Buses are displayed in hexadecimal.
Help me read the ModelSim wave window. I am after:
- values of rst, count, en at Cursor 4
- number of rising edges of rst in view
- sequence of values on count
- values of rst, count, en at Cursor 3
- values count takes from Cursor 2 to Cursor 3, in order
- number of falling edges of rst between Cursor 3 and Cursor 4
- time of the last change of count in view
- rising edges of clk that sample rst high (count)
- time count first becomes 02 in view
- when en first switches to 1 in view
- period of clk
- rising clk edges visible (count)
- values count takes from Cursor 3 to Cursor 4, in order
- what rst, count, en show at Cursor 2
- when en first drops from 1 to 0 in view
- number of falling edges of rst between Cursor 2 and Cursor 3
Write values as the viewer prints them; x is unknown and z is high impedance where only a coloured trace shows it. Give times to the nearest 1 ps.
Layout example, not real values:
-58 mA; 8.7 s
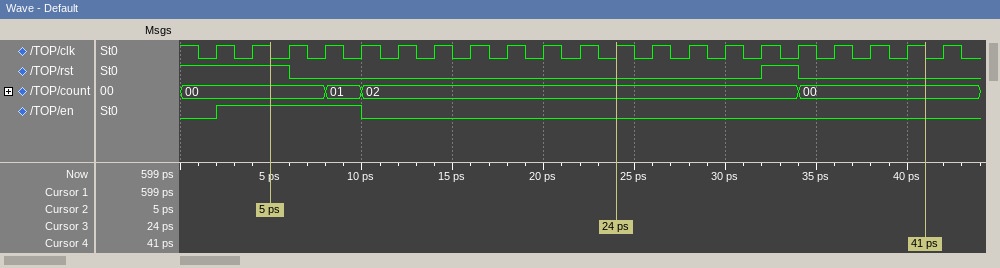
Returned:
rst=0, count=00, en=0; 1; 00, 01, 02, 00; rst=0, count=02, en=0; 00, 01, 02; 1; 34 ps; 4; 10 ps; 2 ps; 2 ps; 21; 02, 00; rst=1, count=00, en=1; 10 ps; 1
